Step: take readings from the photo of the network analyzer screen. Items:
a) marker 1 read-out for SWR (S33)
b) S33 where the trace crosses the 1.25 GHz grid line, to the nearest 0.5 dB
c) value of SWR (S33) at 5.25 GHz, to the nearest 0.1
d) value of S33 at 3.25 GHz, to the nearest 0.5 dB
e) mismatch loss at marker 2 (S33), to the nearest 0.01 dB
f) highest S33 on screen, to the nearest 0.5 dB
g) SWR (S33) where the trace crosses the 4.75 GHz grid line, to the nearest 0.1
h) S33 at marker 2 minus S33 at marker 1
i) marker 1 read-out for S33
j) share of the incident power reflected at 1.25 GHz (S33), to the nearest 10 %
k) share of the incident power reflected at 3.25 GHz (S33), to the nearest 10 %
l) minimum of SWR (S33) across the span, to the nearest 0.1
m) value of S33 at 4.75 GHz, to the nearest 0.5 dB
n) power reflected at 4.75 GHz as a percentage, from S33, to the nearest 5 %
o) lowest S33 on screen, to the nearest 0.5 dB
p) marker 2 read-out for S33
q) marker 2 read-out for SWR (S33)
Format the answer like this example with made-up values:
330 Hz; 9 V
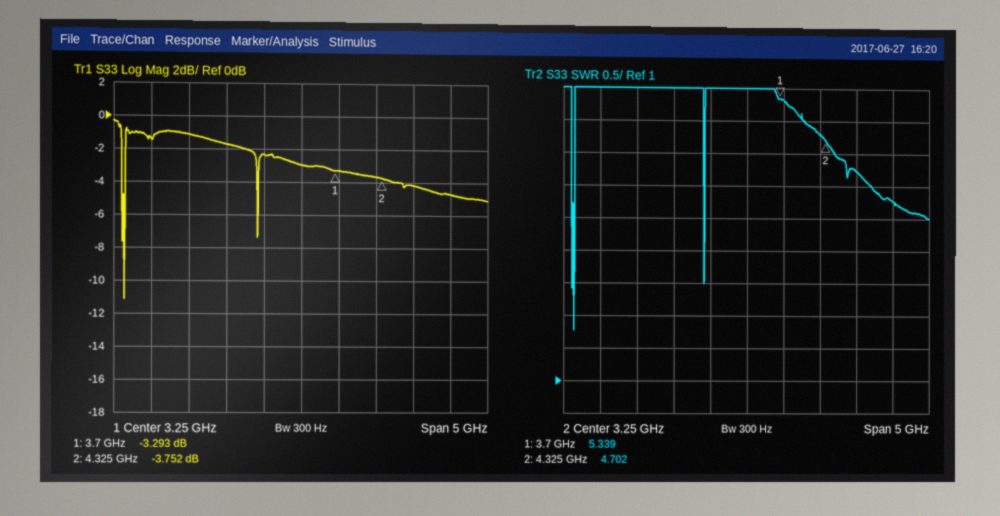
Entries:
5.339; -1.5 dB; 3.8; -3.0 dB; 2.38 dB; -0.5 dB; 4.2; -0.459 dB; -3.293 dB; 70 %; 50 %; 1.8; -4.0 dB; 40 %; -11.0 dB; -3.752 dB; 4.702
